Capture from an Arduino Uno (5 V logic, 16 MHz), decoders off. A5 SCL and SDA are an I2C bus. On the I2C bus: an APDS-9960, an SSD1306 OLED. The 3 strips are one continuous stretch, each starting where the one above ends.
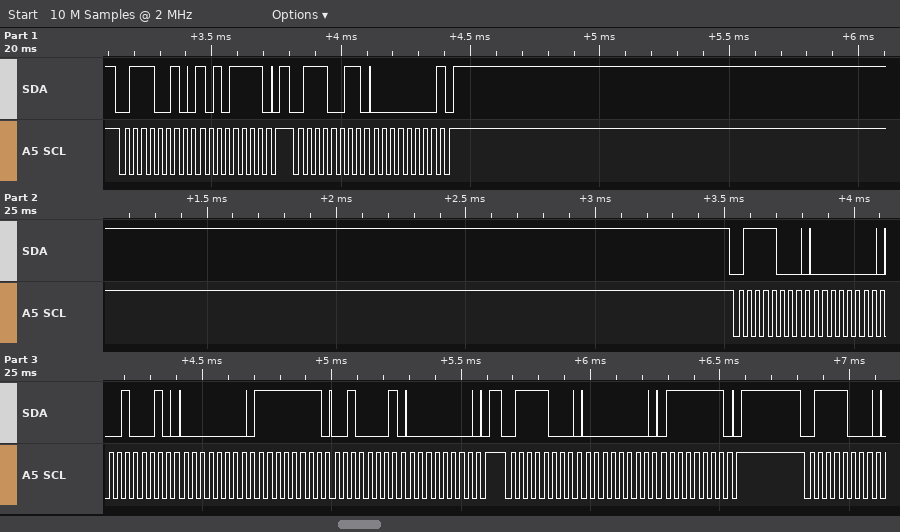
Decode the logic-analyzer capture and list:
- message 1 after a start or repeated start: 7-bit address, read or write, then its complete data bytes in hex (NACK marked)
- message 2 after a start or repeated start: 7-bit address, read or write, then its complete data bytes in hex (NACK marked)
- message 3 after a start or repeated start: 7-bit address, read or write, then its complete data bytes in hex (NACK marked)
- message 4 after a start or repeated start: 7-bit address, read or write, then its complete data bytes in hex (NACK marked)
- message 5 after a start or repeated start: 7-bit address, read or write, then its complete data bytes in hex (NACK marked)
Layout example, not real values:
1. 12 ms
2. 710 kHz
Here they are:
1. 0x39 write: AF
2. 0x39 read: 00 NACK
3. 0x3C write: 00 22 00 FF 21 00
4. 0x3C write: 00 7F
5. 0x3C write
